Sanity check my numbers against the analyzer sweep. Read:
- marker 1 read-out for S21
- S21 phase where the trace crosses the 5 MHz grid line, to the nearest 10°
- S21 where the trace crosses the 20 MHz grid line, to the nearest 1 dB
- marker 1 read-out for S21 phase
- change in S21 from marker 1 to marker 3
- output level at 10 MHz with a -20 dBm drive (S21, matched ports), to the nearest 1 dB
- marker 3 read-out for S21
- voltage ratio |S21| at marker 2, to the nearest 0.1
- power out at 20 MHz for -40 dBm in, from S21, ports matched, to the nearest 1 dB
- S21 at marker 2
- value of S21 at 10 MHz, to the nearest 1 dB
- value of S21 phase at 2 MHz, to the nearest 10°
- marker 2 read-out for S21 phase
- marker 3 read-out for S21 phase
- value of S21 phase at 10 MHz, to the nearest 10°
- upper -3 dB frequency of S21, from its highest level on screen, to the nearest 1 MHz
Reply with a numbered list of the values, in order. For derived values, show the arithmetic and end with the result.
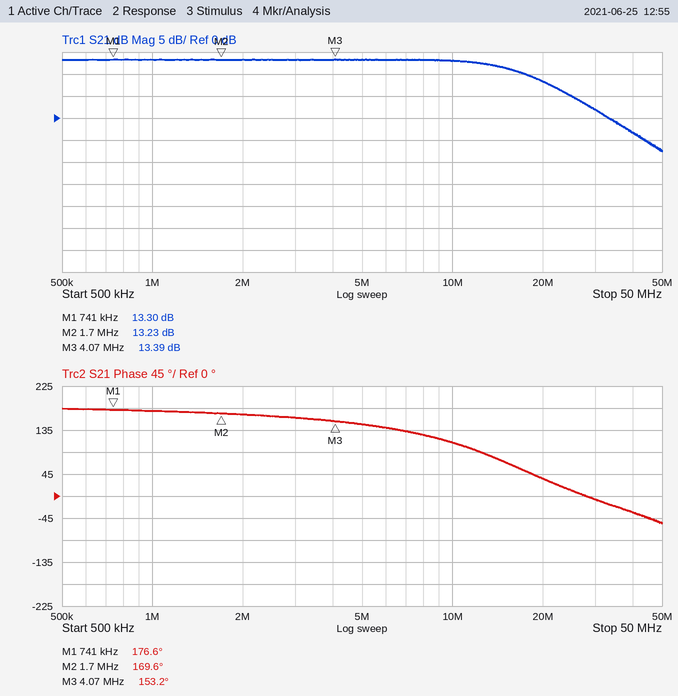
1. 13.30 dB
2. 150°
3. 8 dB
4. 176.6°
5. 13.39 − (13.3) = 0.09 dB
6. -20 dBm + (13 dB) = -7 dBm
7. 13.39 dB
8. 10^(13.23/20) ≈ 4.6
9. -40 dBm + (8 dB) = -32 dBm
10. 13.23 dB
11. 13 dB
12. 170°
13. 169.6°
14. 153.2°
15. 110°
16. 17 MHz
